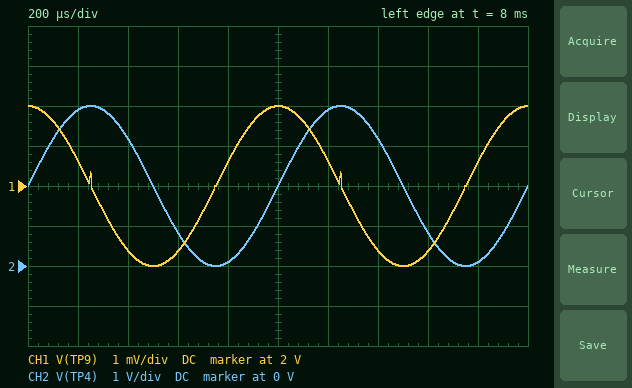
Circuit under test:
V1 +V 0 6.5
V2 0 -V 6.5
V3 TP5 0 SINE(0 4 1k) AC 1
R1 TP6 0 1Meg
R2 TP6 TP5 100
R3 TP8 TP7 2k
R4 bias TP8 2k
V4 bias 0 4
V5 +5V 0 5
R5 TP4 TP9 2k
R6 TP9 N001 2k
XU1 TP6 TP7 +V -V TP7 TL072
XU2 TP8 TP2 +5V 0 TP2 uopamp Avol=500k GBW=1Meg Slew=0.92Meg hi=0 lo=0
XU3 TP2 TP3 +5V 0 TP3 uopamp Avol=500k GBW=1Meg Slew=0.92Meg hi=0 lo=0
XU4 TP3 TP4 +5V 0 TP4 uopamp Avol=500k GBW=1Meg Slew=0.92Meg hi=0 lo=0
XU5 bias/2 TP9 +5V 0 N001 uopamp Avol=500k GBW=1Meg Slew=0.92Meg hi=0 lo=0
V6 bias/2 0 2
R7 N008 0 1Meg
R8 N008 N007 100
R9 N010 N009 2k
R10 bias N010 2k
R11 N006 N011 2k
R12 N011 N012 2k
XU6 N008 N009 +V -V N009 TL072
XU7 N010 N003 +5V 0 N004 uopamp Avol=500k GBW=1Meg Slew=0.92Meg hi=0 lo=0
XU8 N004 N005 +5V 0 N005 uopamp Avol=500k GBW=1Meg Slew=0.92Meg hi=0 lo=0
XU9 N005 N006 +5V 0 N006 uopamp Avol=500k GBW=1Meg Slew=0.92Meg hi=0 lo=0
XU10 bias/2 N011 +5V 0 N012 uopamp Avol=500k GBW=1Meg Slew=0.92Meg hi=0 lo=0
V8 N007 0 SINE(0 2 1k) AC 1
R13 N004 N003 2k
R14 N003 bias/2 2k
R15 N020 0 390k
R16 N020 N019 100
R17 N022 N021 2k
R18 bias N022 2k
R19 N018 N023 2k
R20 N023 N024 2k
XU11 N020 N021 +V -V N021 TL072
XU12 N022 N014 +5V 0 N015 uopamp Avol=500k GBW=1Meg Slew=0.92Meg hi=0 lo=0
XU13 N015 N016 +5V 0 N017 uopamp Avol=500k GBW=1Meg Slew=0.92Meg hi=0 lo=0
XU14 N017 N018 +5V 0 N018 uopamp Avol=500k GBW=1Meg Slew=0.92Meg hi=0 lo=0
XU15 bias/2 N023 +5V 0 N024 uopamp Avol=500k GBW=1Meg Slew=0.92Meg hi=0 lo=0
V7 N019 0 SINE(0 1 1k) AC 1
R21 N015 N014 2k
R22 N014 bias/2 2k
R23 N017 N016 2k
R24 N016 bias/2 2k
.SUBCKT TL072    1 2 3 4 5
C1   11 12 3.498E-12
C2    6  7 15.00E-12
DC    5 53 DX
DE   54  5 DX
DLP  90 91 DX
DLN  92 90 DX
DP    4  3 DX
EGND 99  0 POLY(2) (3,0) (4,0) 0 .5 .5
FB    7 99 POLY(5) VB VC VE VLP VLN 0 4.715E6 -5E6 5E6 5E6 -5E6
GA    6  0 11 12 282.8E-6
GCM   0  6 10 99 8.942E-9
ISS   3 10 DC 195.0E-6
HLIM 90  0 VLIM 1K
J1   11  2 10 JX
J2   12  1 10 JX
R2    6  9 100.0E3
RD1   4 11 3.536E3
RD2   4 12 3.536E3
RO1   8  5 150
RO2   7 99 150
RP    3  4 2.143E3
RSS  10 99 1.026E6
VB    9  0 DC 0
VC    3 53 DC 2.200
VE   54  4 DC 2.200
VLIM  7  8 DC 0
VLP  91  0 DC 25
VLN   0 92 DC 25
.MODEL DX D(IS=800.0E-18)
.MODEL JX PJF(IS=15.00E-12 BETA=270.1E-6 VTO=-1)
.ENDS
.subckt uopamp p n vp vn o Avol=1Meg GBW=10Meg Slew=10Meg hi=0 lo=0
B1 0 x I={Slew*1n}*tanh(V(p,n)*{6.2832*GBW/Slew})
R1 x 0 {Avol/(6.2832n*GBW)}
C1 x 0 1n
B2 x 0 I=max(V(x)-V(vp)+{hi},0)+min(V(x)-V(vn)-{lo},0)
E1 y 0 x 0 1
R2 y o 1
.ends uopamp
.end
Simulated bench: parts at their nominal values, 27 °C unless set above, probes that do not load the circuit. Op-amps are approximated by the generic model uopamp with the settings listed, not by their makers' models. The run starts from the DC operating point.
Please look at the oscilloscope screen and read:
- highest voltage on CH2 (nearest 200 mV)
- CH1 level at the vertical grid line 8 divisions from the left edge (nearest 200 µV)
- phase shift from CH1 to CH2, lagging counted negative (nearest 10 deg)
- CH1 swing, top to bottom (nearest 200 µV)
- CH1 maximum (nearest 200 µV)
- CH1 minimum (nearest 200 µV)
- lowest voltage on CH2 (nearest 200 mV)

4.0 V
1.9984 V
-90 deg
4.0 mV
2.0020 V
1.9980 V
0 V
